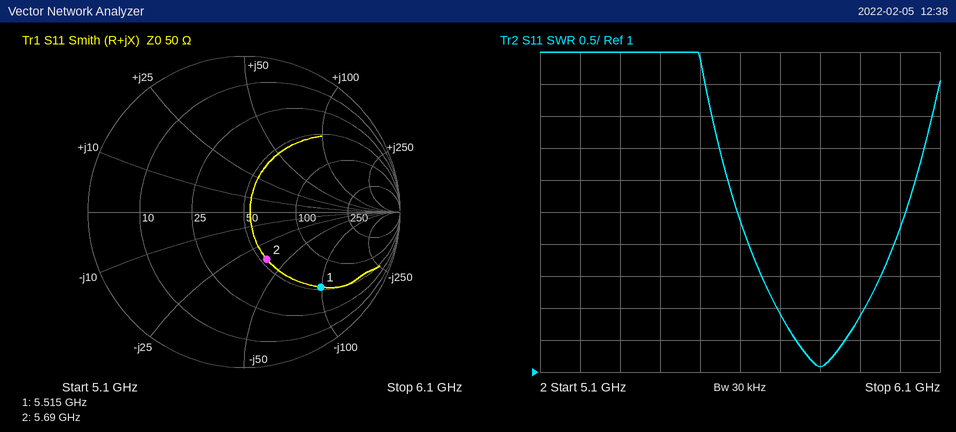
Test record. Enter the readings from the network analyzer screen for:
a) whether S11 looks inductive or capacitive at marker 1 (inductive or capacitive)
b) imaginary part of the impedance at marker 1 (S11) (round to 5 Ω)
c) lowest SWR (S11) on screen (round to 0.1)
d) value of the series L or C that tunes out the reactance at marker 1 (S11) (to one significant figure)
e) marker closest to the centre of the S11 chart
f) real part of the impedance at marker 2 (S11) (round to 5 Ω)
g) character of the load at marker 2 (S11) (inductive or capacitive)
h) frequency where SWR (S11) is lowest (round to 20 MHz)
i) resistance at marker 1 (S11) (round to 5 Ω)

capacitive
-100 Ω
1.1
3 nH
marker 2
55 Ω
capacitive
5.80 GHz
55 Ω
